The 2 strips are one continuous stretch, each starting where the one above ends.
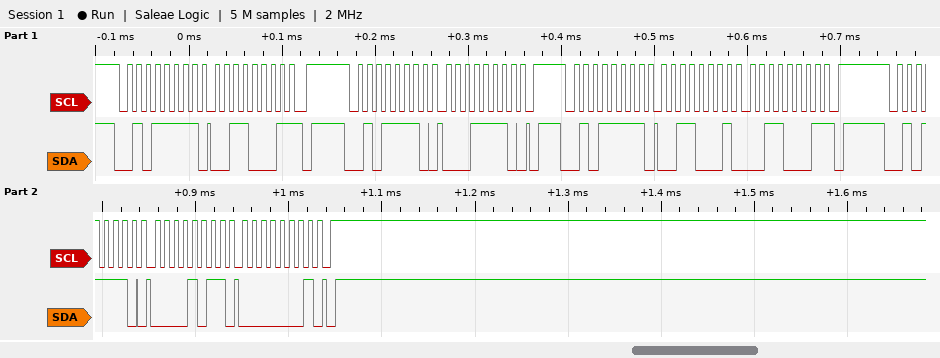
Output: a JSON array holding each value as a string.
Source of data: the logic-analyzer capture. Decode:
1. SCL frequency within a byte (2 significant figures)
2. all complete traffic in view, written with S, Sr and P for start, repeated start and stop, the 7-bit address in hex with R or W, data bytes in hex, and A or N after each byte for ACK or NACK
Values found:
["100 kHz", "S 2FR A 31 N P S 2FW A 1E A P S 2FR A 31 A 31 N P S 2FW A 0B A 01 A P"]
